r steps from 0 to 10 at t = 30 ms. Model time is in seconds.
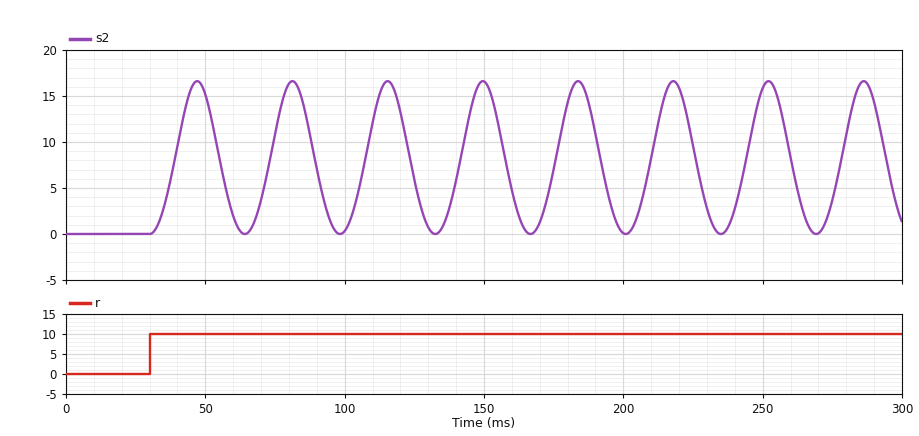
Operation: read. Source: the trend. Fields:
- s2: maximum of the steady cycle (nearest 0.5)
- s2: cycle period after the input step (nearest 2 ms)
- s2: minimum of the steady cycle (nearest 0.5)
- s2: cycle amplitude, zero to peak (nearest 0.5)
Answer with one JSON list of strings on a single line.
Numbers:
["16.5", "34 ms", "0.0", "8.5"]
